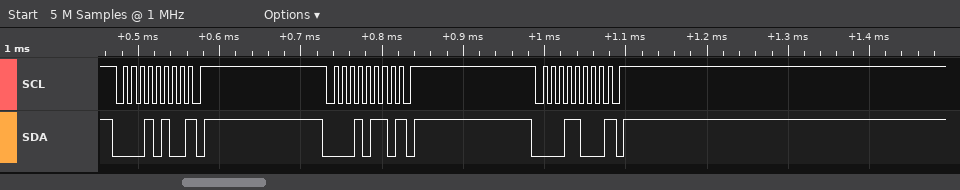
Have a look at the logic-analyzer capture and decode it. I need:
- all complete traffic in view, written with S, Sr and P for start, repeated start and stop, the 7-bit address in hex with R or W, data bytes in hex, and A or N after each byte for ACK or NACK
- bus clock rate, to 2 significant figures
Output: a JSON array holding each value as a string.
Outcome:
["S 0AW N P S 0BW N P S 0CW N P", "100 kHz"]
